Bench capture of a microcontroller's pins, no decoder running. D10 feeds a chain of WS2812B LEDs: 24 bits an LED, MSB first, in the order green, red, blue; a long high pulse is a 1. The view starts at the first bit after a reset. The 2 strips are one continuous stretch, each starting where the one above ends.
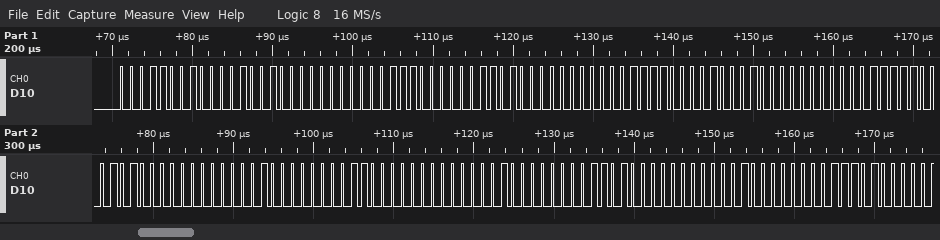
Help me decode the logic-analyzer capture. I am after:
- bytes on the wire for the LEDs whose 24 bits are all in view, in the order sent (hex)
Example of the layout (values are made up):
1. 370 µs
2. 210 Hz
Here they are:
1. 19 09 00 1C 0D 00 1E 11 00 1F 14 00 20 18 00 20 1A 00
